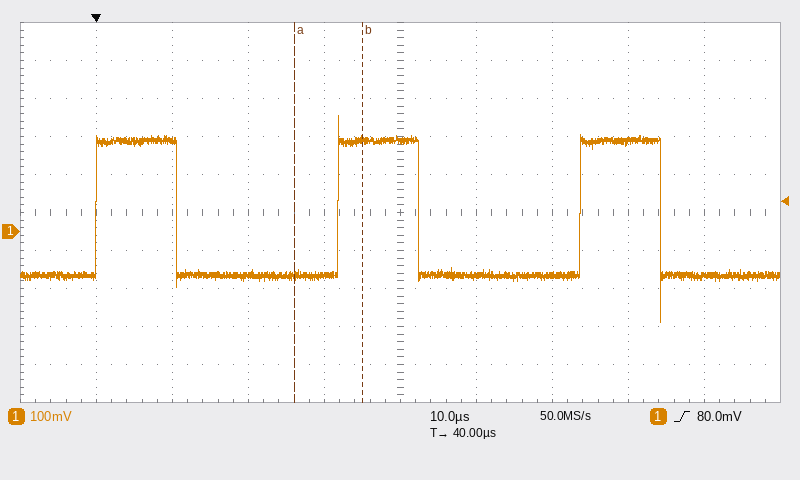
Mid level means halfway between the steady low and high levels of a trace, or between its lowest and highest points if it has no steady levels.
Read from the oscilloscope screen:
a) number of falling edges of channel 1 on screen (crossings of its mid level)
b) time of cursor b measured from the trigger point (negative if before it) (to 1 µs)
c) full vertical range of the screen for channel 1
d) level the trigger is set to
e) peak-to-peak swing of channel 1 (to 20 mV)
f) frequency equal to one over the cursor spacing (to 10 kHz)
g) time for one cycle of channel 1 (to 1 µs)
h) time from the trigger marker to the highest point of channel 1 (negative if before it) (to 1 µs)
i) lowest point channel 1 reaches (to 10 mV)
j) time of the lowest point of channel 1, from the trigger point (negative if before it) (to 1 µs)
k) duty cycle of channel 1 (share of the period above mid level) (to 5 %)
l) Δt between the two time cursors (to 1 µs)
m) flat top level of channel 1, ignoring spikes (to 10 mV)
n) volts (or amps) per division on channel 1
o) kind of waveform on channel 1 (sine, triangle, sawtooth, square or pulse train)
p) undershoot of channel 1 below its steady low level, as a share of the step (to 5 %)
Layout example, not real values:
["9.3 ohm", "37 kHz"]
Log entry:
["3", "+35 µs", "1 V", "80.0 mV", "540 mV", "110 kHz", "32 µs", "+32 µs", "-240 mV", "+74 µs", "35 %", "9 µs", "240 mV", "100 mV", "pulse train", "35 %"]
